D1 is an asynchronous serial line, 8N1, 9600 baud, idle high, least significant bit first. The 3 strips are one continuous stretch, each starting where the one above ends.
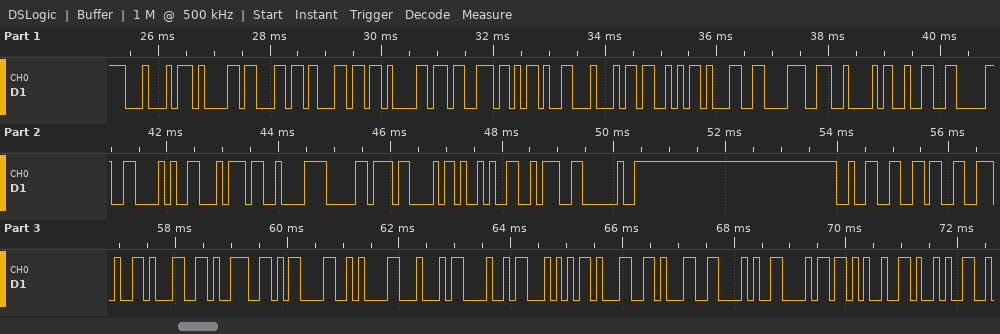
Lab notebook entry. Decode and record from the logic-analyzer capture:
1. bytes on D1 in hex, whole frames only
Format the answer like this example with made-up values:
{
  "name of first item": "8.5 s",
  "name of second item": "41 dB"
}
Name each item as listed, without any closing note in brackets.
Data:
{
  "bytes on D1 in hex, whole frames only": "44 61 6C 6C 61 73 2D 44 53 31 38 42 32 30 28 74 C2 B0 43 29 3A 20 32 36 2E 31 39 0D 0A 44 48 54 31 31 28 68 25 29"
}
